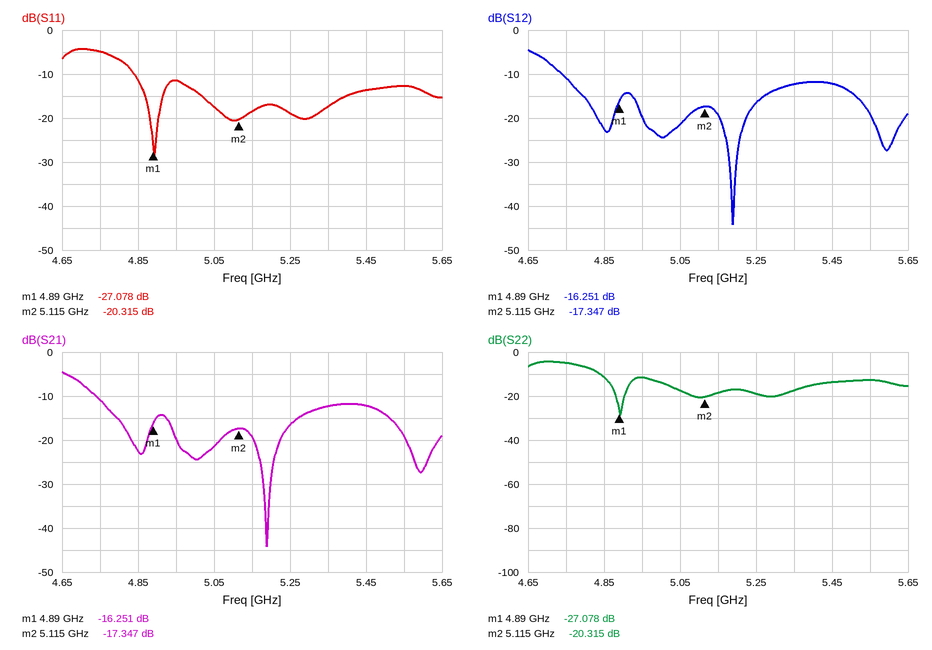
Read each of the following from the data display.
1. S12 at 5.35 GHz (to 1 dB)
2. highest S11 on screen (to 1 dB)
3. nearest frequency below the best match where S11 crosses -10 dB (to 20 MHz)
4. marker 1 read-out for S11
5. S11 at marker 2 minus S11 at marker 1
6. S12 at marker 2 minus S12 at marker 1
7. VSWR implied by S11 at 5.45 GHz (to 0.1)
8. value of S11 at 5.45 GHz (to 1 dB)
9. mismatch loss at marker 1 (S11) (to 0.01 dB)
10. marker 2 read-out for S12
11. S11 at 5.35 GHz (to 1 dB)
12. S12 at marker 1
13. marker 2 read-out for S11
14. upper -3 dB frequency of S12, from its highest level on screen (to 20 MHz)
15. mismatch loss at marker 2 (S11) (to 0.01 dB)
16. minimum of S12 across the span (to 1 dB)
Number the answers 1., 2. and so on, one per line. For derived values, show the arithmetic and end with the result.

1. -12 dB
2. -4 dB
3. 4.84 GHz
4. -27.078 dB
5. -20.315 − (-27.078) = 6.763 dB
6. -17.347 − (-16.251) = -1.096 dB
7. |Γ| = 10^(-14/20) = 0.1995; VSWR = (1 + 0.1995)/(1 − 0.1995) ≈ 1.5
8. -14 dB
9. −10 log10(1 − 10^(-27.078/10)) ≈ 0.01 dB
10. -17.347 dB
11. -17 dB
12. -16.251 dB
13. -20.315 dB
14. 4.70 GHz
15. −10 log10(1 − 10^(-20.315/10)) ≈ 0.04 dB
16. -44 dB
